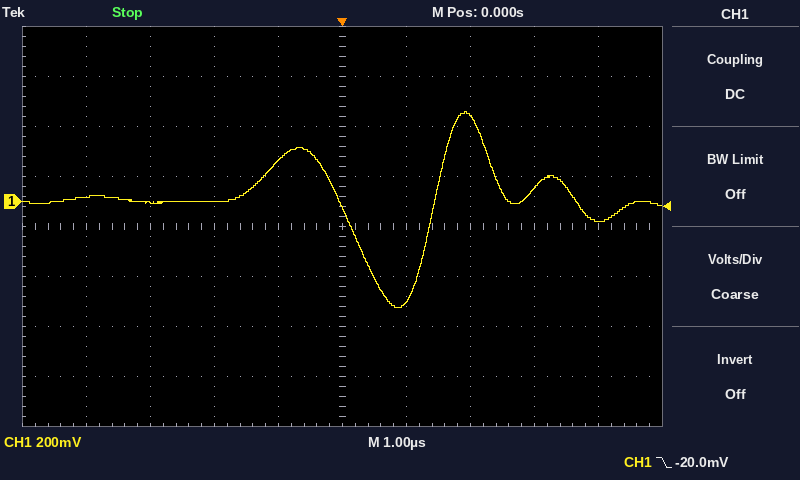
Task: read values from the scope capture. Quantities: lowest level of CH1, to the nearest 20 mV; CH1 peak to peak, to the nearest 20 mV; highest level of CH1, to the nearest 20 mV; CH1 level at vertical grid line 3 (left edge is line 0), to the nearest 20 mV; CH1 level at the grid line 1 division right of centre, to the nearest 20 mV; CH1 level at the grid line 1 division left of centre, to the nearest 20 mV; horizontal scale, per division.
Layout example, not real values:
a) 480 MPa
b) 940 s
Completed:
a) -420 mV
b) 780 mV
c) 360 mV
d) 0 mV
e) -400 mV
f) 160 mV
g) 1 µs
